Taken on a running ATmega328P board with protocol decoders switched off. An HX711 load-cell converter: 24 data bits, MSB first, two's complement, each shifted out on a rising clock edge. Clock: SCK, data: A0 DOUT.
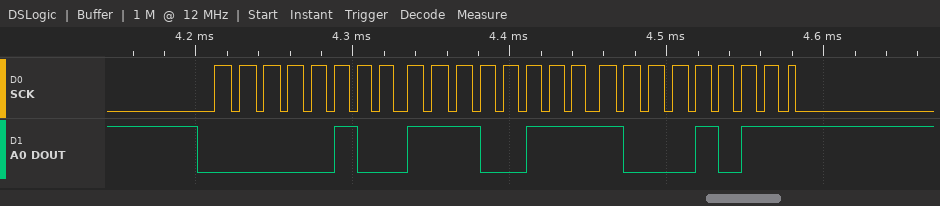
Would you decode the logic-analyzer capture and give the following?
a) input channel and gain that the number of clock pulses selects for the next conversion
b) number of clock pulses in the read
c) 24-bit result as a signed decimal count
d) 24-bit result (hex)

channel A, gain 128
25
321419
0x04E78B
